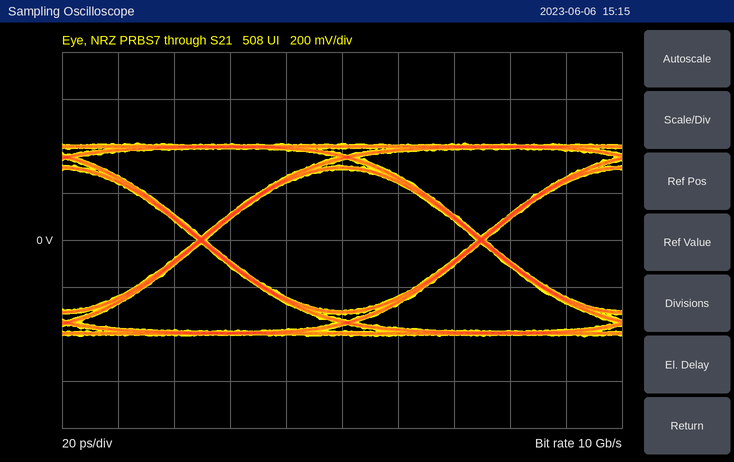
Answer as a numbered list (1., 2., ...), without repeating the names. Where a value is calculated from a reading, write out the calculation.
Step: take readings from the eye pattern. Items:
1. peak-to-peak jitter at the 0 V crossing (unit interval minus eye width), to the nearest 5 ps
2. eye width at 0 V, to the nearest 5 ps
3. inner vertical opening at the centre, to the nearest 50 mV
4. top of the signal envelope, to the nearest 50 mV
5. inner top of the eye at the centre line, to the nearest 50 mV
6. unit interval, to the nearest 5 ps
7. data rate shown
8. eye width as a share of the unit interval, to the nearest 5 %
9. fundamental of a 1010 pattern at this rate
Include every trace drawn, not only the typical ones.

1. 5 ps
2. 95 ps
3. 600 mV
4. 400 mV
5. 300 mV
6. 100 ps
7. 10 Gb/s
8. 95 ps / 100 ps ≈ 95 %
9. 5 GHz
